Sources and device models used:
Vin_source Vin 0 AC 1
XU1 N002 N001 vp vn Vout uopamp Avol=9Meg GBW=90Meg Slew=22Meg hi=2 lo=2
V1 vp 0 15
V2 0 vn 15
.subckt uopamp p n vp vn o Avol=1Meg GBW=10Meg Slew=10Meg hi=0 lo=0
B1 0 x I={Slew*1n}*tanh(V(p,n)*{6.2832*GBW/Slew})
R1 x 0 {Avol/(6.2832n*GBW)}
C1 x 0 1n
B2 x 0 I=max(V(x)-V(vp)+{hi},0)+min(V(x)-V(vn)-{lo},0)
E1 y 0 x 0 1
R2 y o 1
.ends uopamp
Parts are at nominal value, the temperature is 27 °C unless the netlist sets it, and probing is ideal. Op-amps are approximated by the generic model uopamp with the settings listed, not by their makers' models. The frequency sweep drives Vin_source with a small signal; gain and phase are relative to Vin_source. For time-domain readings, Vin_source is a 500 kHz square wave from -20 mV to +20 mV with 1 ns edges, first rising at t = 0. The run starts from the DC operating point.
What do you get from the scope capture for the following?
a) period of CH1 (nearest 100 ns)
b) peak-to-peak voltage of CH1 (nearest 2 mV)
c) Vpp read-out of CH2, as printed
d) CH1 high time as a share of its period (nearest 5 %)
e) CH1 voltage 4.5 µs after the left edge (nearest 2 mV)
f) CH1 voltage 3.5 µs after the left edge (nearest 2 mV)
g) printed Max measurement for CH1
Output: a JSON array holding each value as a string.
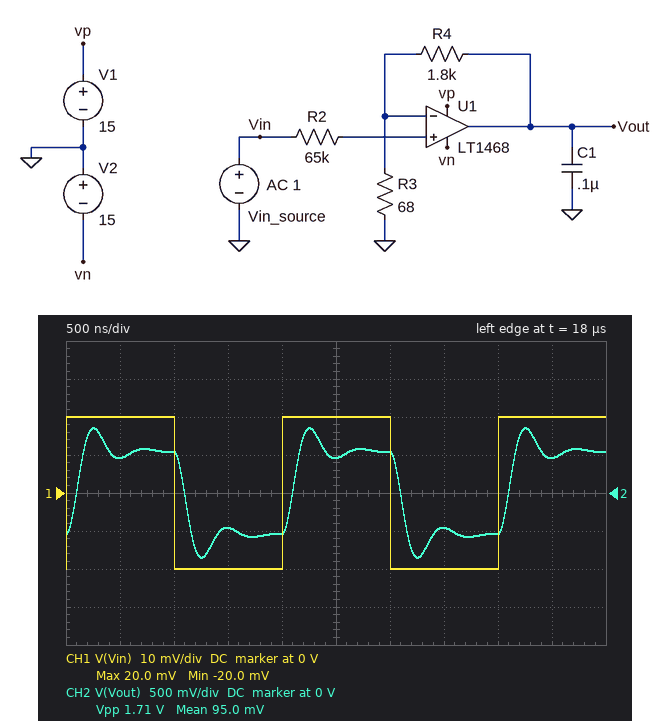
["2.0 µs", "40 mV", "1.71 V", "50 %", "20 mV", "-20 mV", "20.0 mV"]
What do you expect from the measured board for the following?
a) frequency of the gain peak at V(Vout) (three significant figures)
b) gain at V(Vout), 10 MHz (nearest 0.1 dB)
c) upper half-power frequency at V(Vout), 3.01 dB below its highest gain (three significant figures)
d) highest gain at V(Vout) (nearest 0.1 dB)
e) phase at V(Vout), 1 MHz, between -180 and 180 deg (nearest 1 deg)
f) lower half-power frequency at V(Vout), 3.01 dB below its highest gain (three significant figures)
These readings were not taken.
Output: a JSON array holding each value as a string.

["1.99 MHz", "3.5 dB", "2.71 MHz", "32.5 dB", "-21 deg", "734 kHz"]
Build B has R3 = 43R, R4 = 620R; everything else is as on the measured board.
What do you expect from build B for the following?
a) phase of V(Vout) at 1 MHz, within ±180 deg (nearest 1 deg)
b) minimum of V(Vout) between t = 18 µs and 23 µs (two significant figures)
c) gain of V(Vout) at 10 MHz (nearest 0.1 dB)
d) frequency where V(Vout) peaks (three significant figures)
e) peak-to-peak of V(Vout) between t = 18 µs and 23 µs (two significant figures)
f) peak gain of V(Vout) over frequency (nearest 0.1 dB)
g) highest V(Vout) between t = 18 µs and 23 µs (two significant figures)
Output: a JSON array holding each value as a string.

["-11 deg", "-550 mV", "3.8 dB", "2.83 MHz", "1.1 V", "29.7 dB", "550 mV"]
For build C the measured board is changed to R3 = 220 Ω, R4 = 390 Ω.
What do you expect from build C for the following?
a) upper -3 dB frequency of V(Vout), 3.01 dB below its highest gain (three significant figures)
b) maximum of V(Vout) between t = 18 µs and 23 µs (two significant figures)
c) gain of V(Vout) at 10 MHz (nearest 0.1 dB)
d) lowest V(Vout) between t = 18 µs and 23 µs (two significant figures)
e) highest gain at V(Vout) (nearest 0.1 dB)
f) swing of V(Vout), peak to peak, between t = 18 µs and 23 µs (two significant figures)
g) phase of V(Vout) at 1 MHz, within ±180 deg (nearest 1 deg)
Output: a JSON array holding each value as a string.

["7.86 MHz", "130 mV", "9.0 dB", "-130 mV", "22.0 dB", "260 mV", "-2 deg"]
